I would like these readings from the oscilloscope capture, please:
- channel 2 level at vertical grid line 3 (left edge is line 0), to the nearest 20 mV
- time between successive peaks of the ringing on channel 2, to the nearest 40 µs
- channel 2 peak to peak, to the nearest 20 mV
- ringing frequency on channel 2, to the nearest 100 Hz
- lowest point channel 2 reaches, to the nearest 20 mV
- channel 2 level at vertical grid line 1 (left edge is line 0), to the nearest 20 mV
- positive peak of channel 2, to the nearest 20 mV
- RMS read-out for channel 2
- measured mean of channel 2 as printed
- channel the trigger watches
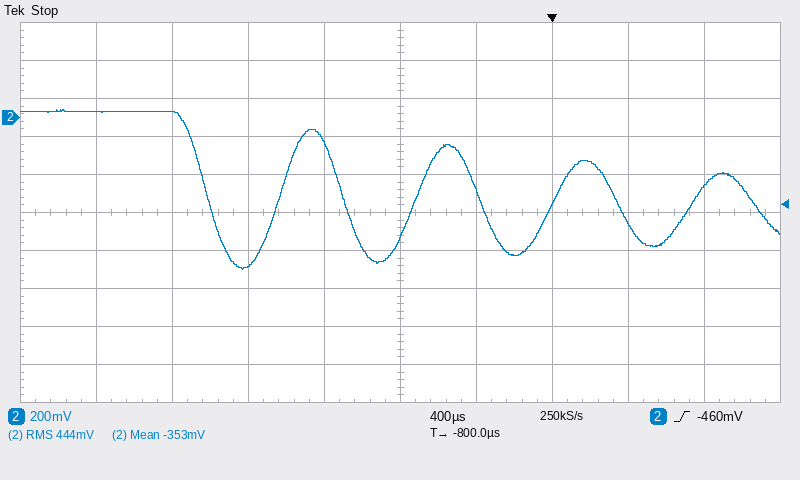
-780 mV
720 µs
840 mV
1.4 kHz
-800 mV
40 mV
40 mV
444 mV
-353 mV
channel 2
